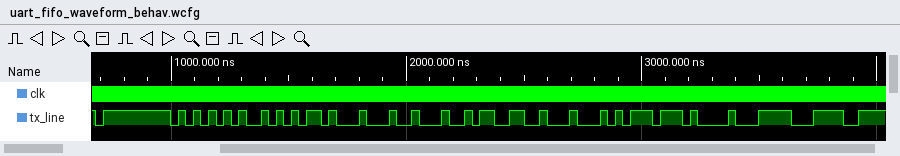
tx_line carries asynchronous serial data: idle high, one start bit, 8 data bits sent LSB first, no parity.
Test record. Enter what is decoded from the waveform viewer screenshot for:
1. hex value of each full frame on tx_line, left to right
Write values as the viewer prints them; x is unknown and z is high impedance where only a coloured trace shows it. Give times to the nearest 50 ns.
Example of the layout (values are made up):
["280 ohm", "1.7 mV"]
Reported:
["FF, 55, AA, 11, 22, 33, 44, 77, 88, 3C"]
